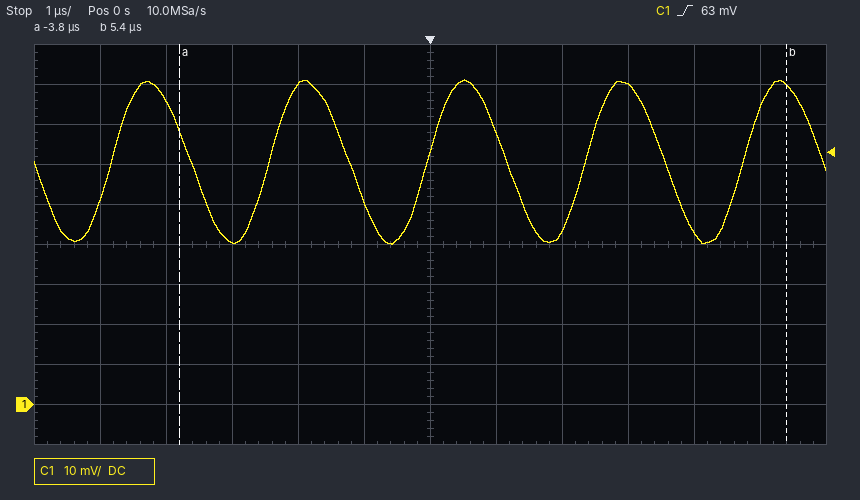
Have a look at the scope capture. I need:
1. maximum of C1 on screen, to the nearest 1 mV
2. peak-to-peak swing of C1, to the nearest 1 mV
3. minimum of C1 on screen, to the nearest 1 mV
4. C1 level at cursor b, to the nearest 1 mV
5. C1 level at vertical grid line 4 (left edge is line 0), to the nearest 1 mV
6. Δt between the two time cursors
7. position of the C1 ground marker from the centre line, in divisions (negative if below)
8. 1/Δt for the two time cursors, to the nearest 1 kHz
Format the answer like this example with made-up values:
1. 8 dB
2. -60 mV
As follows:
1. 81 mV
2. 41 mV
3. 40 mV
4. 80 mV
5. 80 mV
6. 9.2 µs
7. -4.0 div
8. 109 kHz
